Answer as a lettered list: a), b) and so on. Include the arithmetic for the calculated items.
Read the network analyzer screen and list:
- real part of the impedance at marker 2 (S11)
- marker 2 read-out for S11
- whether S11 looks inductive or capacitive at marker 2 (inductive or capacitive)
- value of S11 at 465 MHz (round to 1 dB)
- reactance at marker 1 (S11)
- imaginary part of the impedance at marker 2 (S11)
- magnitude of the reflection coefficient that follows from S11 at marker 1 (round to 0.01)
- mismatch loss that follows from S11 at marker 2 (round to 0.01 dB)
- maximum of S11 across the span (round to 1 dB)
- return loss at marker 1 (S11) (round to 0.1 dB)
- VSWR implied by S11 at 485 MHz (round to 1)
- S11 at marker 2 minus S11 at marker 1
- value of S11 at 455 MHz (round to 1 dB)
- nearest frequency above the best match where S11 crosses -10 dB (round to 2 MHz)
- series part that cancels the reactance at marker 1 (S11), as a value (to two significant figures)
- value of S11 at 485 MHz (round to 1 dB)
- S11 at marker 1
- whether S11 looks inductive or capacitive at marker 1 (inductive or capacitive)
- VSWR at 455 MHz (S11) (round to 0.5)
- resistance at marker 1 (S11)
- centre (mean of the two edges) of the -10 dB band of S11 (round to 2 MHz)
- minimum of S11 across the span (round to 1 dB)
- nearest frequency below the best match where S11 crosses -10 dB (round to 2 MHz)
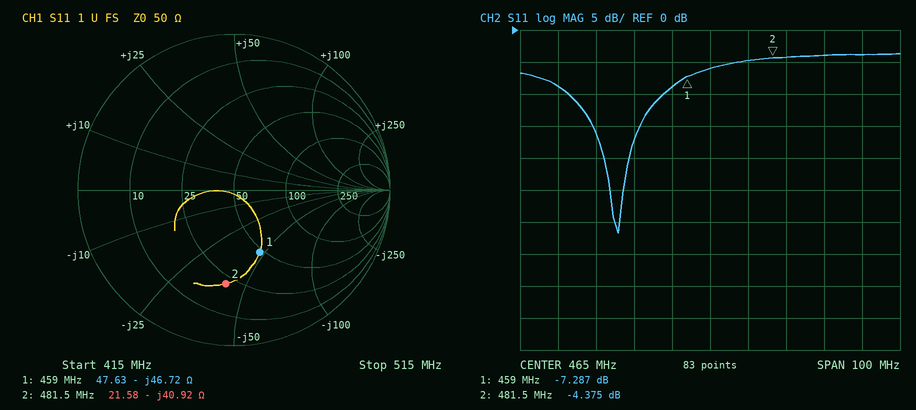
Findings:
a) 21.58 Ω
b) -4.375 dB
c) capacitive
d) -6 dB
e) -46.72 Ω
f) -40.92 Ω
g) 10^(-7.287/20) ≈ 0.43
h) −10 log10(1 − 10^(-4.375/10)) ≈ 1.97 dB
i) -4 dB
j) 7.3 dB
k) |Γ| = 10^(-4/20) = 0.6310; VSWR = (1 + 0.6310)/(1 − 0.6310) ≈ 4
l) -4.375 − (-7.287) = 2.912 dB
m) -9 dB
n) 452 MHz
o) L = 46.72 Ω/(2π × 459 MHz) ≈ 16 nH
p) -4 dB
q) -7.287 dB
r) capacitive
s) |Γ| = 10^(-9/20) = 0.3548; VSWR = (1 + 0.3548)/(1 − 0.3548) ≈ 2.10, so 2.0 to the nearest 0.5
t) 47.63 Ω
u) 440 MHz
v) -32 dB
w) 428 MHz
